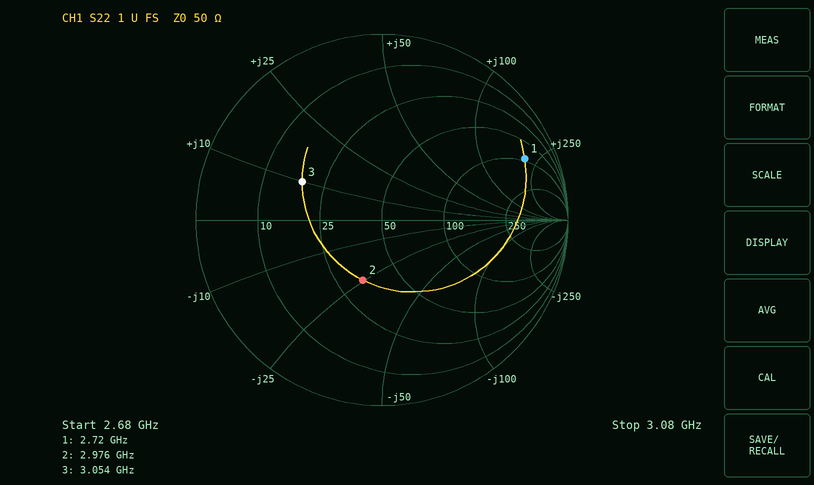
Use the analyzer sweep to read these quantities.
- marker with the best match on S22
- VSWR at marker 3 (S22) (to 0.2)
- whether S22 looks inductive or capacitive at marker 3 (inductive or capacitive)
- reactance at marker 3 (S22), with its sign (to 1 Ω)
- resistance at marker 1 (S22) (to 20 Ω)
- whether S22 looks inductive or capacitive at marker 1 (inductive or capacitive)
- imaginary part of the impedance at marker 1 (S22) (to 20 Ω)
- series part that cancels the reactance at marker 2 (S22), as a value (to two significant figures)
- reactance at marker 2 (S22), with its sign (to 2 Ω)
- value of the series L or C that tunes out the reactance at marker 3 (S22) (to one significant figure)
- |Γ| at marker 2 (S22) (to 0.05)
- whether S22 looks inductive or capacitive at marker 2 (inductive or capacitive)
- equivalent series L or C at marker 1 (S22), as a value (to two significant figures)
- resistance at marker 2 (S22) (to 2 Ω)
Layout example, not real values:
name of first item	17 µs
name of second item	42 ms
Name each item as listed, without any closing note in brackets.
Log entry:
marker with the best match on S22	marker 2
VSWR at marker 3 (S22)	2.8
whether S22 looks inductive or capacitive at marker 3	inductive
reactance at marker 3 (S22), with its sign	+10 Ω
resistance at marker 1 (S22)	100 Ω
whether S22 looks inductive or capacitive at marker 1	inductive
imaginary part of the impedance at marker 1 (S22)	+200 Ω
series part that cancels the reactance at marker 2 (S22), as a value	1.3 nH
reactance at marker 2 (S22), with its sign	-24 Ω
value of the series L or C that tunes out the reactance at marker 3 (S22)	5 pF
|Γ| at marker 2 (S22)	0.35
whether S22 looks inductive or capacitive at marker 2	capacitive
equivalent series L or C at marker 1 (S22), as a value	12 nH
resistance at marker 2 (S22)	34 Ω
